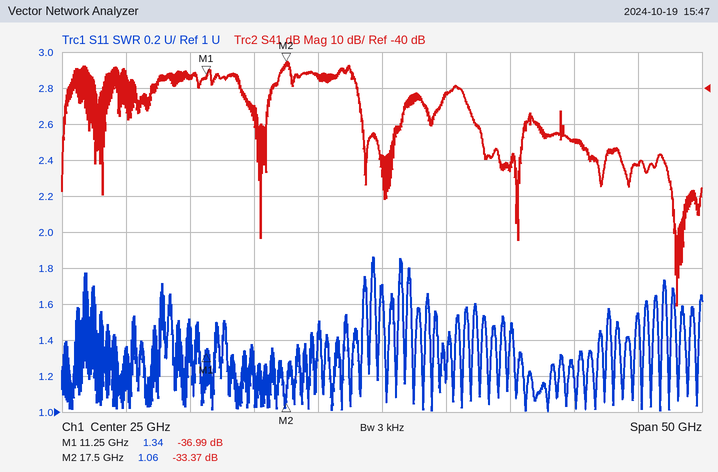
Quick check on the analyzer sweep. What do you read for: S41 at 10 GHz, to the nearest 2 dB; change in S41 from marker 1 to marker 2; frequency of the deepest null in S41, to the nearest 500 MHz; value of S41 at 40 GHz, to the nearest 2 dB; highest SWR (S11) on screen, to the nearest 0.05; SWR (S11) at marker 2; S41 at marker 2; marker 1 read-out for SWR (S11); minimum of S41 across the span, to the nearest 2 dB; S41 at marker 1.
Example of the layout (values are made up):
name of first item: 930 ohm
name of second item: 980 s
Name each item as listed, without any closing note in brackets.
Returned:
S41 at 10 GHz, to the nearest 2 dB: -36 dB
change in S41 from marker 1 to marker 2: 3.62 dB
frequency of the deepest null in S41, to the nearest 500 MHz: 48.0 GHz
value of S41 at 40 GHz, to the nearest 2 dB: -54 dB
highest SWR (S11) on screen, to the nearest 0.05: 1.85
SWR (S11) at marker 2: 1.06
S41 at marker 2: -33.37 dB
marker 1 read-out for SWR: 1.34
minimum of S41 across the span, to the nearest 2 dB: -100 dB
S41 at marker 1: -36.99 dB
